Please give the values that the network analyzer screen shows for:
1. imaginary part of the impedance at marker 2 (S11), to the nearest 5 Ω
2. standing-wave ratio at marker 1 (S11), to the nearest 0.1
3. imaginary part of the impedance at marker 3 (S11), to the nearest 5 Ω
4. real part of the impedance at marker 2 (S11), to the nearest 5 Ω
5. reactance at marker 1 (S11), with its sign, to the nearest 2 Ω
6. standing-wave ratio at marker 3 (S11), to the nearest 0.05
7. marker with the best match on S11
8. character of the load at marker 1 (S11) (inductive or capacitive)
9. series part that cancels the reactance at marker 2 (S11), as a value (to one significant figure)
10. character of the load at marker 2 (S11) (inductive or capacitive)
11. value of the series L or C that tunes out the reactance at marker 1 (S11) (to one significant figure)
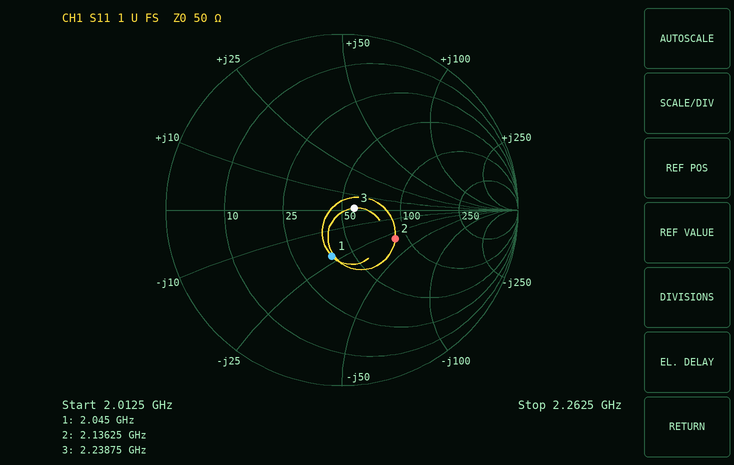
-30 Ω
1.7
0 Ω
85 Ω
-22 Ω
1.15
marker 3
capacitive
2 nH
capacitive
2 nH
